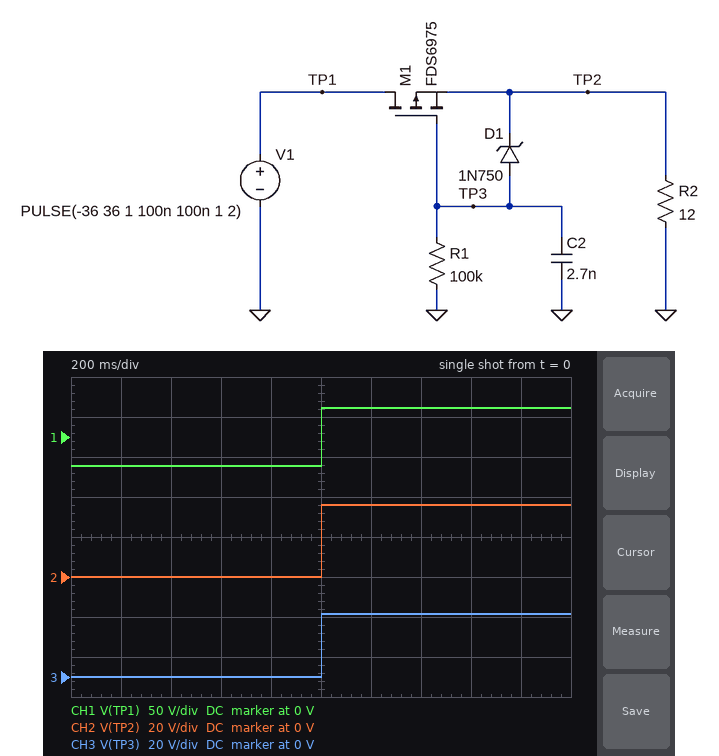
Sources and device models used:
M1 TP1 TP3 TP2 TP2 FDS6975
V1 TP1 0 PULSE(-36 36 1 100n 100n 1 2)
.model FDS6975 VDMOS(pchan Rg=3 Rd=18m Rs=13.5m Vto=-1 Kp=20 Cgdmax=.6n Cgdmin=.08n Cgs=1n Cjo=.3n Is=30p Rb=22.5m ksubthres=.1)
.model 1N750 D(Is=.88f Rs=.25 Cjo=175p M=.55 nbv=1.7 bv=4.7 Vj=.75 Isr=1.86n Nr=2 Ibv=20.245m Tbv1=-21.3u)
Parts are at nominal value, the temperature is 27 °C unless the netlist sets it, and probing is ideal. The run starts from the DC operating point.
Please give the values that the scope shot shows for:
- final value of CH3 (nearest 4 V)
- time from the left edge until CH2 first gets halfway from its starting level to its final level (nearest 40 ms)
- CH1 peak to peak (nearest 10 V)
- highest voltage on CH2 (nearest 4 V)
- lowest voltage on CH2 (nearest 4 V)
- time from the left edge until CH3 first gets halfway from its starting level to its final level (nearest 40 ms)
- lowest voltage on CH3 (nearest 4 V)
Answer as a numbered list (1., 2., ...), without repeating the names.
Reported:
1. 32 V
2. 1.00 s
3. 70 V
4. 36 V
5. 0 V
6. 1.00 s
7. 0 V
